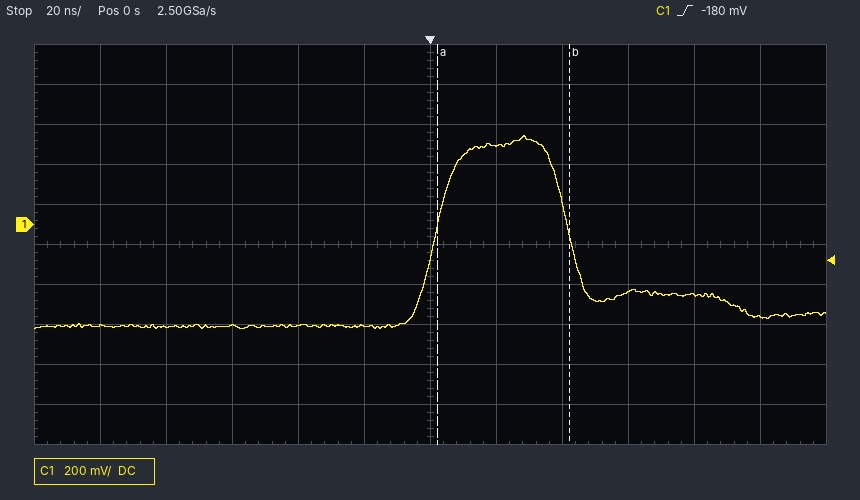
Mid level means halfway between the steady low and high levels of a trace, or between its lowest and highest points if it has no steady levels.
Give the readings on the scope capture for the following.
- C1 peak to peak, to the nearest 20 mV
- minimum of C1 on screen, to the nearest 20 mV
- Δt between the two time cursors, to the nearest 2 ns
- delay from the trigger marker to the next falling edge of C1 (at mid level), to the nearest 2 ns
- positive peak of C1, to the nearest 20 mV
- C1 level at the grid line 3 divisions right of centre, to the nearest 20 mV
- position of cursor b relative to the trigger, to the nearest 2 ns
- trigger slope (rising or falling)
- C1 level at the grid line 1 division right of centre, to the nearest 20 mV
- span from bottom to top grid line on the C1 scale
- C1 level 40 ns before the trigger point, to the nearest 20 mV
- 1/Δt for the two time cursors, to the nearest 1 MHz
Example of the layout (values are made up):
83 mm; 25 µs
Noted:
960 mV; -520 mV; 40 ns; 42 ns; 440 mV; -340 mV; +42 ns; rising; 400 mV; 2 V; -500 mV; 25 MHz
